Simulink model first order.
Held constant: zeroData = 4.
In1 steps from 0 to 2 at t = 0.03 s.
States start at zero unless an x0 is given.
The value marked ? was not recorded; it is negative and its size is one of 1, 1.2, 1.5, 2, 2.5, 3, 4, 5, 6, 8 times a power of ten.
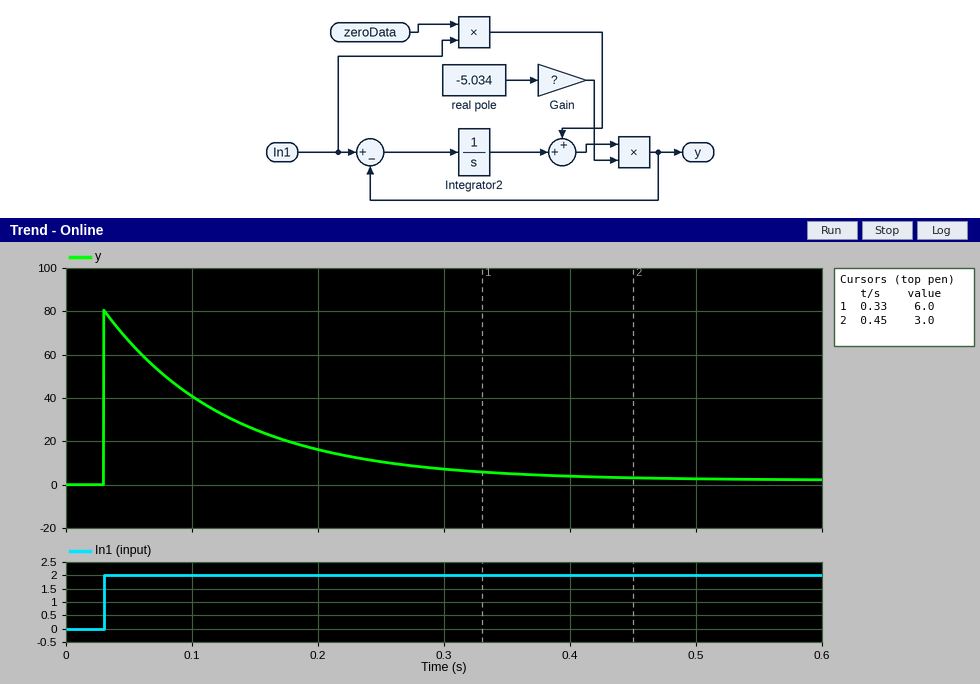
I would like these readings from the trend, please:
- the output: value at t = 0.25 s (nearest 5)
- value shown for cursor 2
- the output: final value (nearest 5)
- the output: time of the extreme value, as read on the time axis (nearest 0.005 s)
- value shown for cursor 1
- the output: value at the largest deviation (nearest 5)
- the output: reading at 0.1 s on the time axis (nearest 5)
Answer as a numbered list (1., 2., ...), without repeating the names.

1. 10
2. 3.0
3. 0
4. 0.030 s
5. 6.0
6. 80
7. 40
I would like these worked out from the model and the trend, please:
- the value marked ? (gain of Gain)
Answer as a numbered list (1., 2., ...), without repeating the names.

1. -2
